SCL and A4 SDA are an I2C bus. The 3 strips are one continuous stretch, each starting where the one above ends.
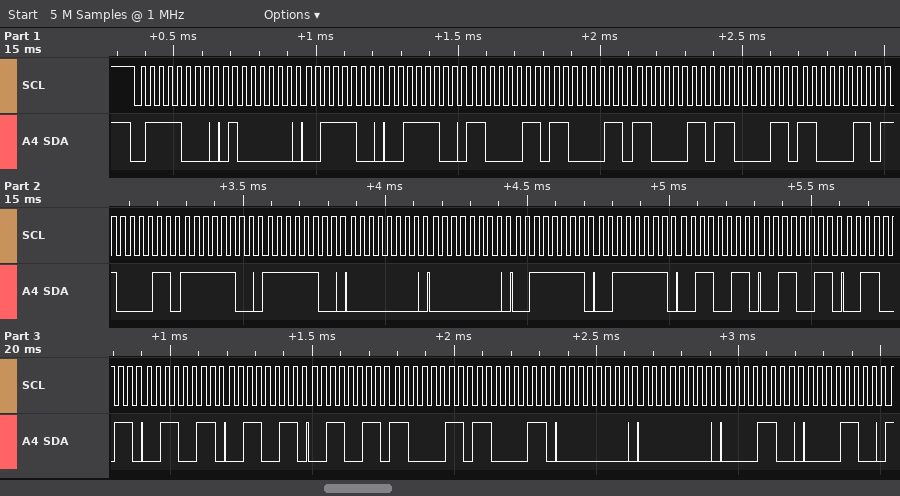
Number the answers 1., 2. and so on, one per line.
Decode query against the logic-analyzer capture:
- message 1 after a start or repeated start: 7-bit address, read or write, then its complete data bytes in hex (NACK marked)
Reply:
1. 0x3C write: 40 3C 3C C3 C3 C3 C3 C3 C3 FC FC 00 00 3F 3F 33 33 33 33 33 33 C3 C3 00 00 0C 0C
